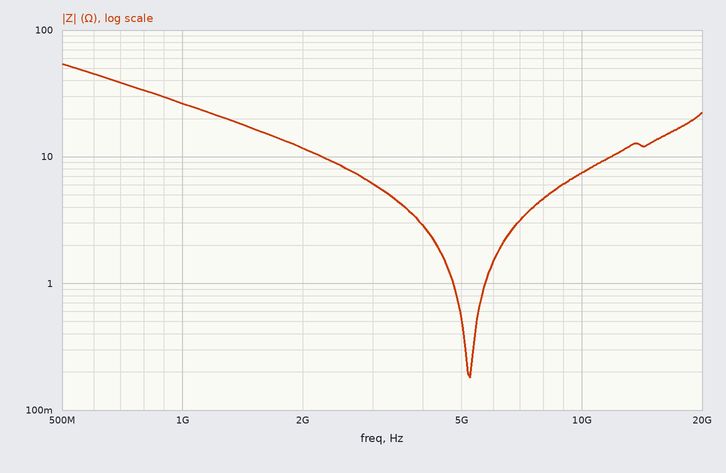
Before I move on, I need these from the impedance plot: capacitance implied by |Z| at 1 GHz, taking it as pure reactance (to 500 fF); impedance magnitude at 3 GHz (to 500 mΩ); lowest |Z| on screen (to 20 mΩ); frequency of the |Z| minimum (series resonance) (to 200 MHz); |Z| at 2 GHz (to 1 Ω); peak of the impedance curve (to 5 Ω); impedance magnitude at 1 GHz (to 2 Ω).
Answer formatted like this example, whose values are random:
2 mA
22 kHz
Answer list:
6.0 pF
6.0 Ω
180 mΩ
5.2 GHz
12 Ω
55 Ω
26 Ω
